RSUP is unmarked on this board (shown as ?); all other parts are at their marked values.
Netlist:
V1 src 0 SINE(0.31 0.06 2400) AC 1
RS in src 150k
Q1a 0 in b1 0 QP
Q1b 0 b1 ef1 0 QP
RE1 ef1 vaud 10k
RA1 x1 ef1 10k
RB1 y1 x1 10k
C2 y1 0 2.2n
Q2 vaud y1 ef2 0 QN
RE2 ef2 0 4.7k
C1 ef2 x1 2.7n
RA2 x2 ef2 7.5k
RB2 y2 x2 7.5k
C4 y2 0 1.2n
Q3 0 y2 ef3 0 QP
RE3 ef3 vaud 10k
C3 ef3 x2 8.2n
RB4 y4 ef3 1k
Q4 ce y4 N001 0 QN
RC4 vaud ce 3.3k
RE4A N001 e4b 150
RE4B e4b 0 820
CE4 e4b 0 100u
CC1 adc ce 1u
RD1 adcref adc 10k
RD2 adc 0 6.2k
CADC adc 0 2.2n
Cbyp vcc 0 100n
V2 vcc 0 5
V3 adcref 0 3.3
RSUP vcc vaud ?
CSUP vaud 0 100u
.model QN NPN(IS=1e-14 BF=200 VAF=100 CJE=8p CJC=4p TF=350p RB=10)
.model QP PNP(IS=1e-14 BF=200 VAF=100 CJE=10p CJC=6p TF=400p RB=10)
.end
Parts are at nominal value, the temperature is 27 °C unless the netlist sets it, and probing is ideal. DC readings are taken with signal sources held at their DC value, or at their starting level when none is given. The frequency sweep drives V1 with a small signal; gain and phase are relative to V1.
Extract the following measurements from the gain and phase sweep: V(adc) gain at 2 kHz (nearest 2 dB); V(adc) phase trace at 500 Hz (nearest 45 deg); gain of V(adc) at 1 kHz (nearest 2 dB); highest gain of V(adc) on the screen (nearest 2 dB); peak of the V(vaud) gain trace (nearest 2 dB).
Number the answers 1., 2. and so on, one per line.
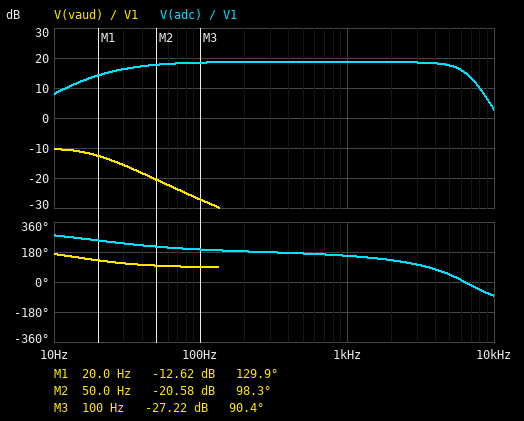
1. 18 dB
2. 180 deg
3. 18 dB
4. 18 dB
5. -10 dB
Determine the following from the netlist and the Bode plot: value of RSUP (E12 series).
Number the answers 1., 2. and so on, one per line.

1. 120 Ω
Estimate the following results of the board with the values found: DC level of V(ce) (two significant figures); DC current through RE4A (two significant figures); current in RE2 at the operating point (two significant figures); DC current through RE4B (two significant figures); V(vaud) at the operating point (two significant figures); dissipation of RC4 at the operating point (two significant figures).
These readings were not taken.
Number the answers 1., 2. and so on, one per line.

1. 2.1 V
2. 820 µA
3. 170 µA
4. 820 µA
5. 4.8 V
6. 2.2 mW
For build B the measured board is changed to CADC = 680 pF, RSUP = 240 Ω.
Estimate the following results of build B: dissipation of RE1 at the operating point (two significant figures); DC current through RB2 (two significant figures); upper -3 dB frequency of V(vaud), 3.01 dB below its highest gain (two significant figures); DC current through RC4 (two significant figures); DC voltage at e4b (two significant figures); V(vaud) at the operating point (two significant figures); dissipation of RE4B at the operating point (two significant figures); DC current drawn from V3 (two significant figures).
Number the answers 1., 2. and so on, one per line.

1. 1.0 mW
2. 1.5 µA
3. 17 Hz
4. 810 µA
5. 670 mV
6. 4.6 V
7. 550 µW
8. 200 µA
